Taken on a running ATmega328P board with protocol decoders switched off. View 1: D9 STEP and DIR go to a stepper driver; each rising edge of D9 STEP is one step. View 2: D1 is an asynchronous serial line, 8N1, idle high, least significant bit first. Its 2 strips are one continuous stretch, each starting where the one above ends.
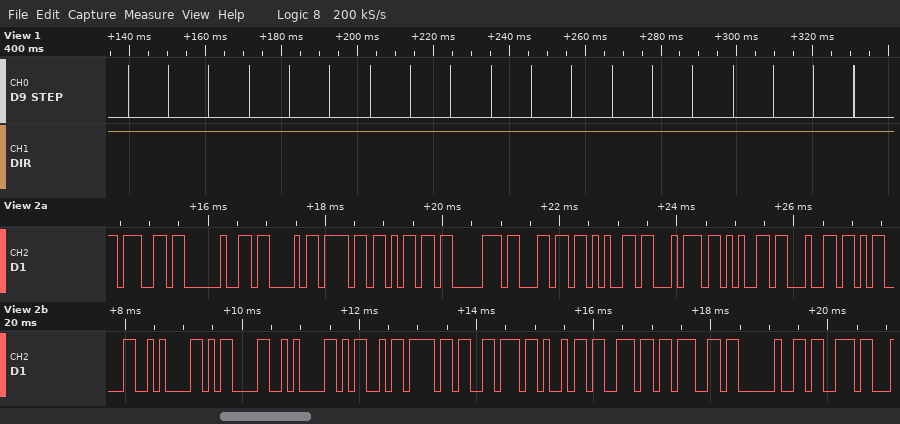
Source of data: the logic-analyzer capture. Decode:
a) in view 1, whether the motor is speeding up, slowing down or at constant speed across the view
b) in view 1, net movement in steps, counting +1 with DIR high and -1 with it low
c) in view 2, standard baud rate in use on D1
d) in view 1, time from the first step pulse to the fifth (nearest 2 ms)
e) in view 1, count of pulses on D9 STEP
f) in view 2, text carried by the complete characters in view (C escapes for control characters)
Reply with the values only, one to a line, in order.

constant speed
+19
9600 baud
42 ms
19
"g Completed\r\n\r\nMoving s"
